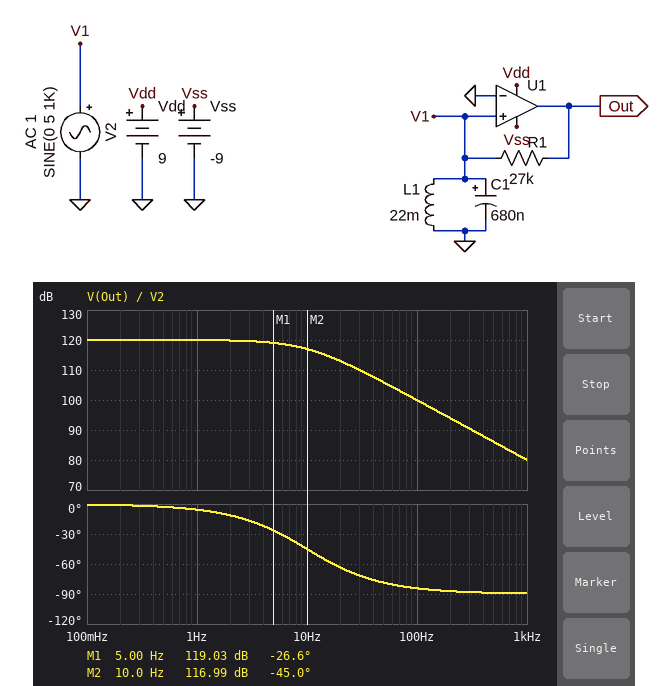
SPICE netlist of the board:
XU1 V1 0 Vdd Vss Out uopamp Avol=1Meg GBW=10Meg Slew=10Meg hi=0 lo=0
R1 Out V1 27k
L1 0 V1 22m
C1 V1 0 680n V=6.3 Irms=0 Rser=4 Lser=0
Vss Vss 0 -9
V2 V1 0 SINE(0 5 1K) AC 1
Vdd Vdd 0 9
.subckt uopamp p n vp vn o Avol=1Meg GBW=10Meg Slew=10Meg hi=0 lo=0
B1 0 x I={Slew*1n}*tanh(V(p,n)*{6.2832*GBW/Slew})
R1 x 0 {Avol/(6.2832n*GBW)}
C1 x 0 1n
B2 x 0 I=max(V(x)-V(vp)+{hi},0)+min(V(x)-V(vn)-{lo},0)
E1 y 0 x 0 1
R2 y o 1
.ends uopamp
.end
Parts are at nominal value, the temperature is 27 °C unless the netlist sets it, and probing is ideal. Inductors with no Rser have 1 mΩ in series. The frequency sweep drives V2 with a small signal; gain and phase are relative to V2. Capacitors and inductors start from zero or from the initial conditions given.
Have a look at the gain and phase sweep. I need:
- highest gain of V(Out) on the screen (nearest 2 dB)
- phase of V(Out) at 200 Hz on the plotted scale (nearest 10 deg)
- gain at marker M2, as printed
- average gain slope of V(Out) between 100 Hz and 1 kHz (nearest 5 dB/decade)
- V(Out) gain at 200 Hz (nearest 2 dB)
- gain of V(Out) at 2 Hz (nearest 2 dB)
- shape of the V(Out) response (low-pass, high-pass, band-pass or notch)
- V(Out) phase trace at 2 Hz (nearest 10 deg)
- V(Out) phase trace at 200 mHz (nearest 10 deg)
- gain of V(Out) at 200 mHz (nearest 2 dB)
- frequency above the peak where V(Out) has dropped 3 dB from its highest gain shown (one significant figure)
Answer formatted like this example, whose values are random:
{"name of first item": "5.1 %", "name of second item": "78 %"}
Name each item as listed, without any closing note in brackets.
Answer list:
{"highest gain of V(Out) on the screen": "120 dB", "phase of V(Out) at 200 Hz on the plotted scale": "-90 deg", "gain at marker M2, as printed": "116.99 dB", "average gain slope of V(Out) between 100 Hz and 1 kHz": "-20 dB/decade", "V(Out) gain at 200 Hz": "94 dB", "gain of V(Out) at 2 Hz": "120 dB", "shape of the V(Out) response": "low-pass", "V(Out) phase trace at 2 Hz": "-10 deg", "V(Out) phase trace at 200 mHz": "0 deg", "gain of V(Out) at 200 mHz": "120 dB", "frequency above the peak where V(Out) has dropped 3 dB from its highest gain shown": "10 Hz"}
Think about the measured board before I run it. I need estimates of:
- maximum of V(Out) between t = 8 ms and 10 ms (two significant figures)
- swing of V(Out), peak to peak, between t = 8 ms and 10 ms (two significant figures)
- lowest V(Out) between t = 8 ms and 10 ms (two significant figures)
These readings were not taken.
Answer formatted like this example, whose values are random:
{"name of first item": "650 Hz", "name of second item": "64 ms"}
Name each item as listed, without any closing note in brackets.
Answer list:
{"maximum of V(Out) between t = 8 ms and 10 ms": "9.0 V", "swing of V(Out), peak to peak, between t = 8 ms and 10 ms": "18 V", "lowest V(Out) between t = 8 ms and 10 ms": "-9.0 V"}
